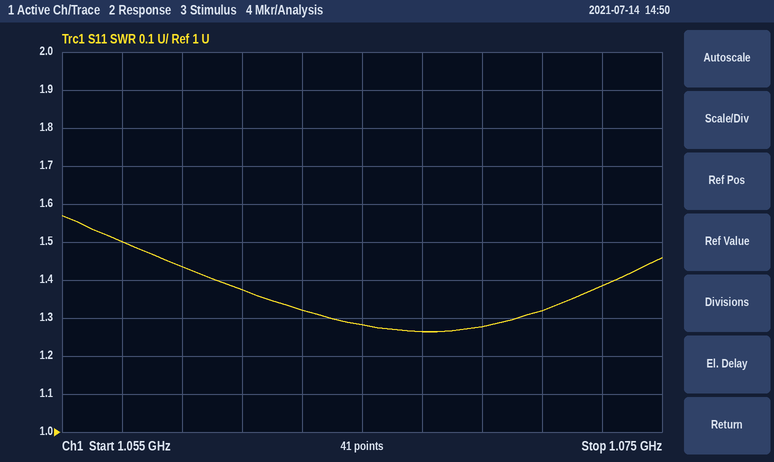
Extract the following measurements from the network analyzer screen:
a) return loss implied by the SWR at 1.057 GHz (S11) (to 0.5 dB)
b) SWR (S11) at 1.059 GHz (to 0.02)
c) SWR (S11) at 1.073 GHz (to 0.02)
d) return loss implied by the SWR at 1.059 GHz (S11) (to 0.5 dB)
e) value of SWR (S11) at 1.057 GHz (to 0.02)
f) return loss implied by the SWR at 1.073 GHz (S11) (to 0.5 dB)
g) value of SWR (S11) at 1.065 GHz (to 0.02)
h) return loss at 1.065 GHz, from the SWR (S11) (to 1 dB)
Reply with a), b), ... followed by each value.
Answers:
a) 14.0 dB
b) 1.44
c) 1.38
d) 15.0 dB
e) 1.50
f) 16.0 dB
g) 1.28
h) 18 dB
